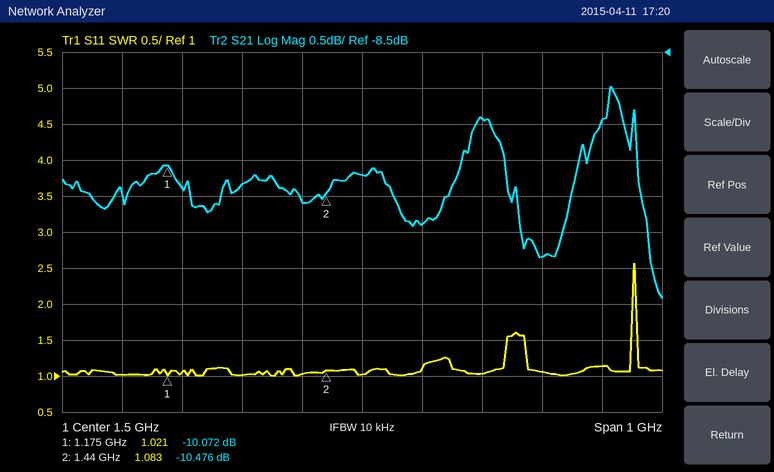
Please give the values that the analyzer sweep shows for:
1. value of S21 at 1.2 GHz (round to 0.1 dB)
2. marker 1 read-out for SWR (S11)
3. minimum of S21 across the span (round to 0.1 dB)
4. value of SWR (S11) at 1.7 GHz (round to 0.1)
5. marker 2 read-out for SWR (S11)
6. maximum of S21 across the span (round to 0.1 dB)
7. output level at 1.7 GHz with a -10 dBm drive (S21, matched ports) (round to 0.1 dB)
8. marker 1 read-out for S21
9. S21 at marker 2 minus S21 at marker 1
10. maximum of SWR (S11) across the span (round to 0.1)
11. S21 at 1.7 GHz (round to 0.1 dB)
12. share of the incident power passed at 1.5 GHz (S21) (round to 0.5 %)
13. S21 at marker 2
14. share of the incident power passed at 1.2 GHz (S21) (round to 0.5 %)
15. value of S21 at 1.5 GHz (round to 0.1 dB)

-10.4 dB
1.021
-11.9 dB
1.0
1.083
-9.0 dB
-19.4 dBm
-10.072 dB
-0.404 dB
2.6
-9.4 dB
9.5 %
-10.476 dB
9.0 %
-10.2 dB
